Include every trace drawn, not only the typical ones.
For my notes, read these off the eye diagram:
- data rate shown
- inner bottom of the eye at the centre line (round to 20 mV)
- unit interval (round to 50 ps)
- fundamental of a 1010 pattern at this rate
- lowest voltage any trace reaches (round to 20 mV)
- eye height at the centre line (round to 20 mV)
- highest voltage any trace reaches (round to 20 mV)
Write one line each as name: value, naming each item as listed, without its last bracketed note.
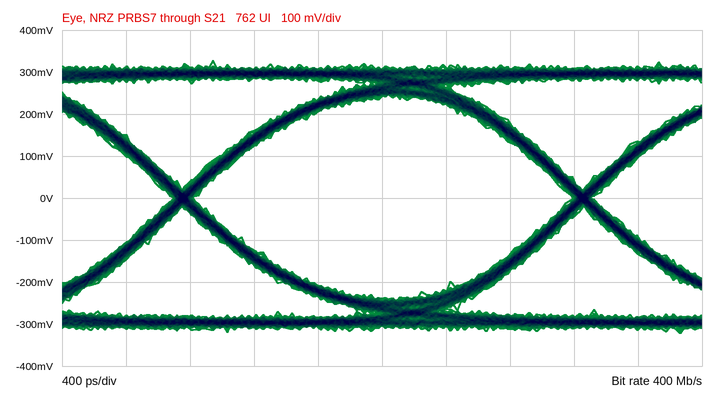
data rate shown: 400 Mb/s
inner bottom of the eye at the centre line: -240 mV
unit interval: 2.50 ns
fundamental of a 1010 pattern at this rate: 200 MHz
lowest voltage any trace reaches: -320 mV
eye height at the centre line: 480 mV
highest voltage any trace reaches: 320 mV
